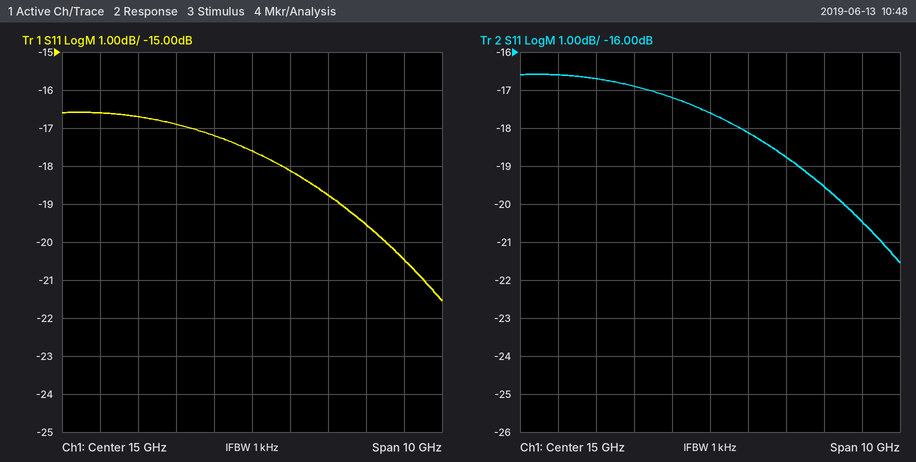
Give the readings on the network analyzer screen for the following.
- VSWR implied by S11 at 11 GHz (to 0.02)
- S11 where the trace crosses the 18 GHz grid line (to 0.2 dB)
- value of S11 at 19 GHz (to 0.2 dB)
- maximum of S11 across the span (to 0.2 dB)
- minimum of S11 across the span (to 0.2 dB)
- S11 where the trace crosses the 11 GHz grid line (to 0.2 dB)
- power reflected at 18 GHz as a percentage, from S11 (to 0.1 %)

1.34
-19.6 dB
-20.4 dB
-16.6 dB
-21.6 dB
-16.6 dB
1.1 %
